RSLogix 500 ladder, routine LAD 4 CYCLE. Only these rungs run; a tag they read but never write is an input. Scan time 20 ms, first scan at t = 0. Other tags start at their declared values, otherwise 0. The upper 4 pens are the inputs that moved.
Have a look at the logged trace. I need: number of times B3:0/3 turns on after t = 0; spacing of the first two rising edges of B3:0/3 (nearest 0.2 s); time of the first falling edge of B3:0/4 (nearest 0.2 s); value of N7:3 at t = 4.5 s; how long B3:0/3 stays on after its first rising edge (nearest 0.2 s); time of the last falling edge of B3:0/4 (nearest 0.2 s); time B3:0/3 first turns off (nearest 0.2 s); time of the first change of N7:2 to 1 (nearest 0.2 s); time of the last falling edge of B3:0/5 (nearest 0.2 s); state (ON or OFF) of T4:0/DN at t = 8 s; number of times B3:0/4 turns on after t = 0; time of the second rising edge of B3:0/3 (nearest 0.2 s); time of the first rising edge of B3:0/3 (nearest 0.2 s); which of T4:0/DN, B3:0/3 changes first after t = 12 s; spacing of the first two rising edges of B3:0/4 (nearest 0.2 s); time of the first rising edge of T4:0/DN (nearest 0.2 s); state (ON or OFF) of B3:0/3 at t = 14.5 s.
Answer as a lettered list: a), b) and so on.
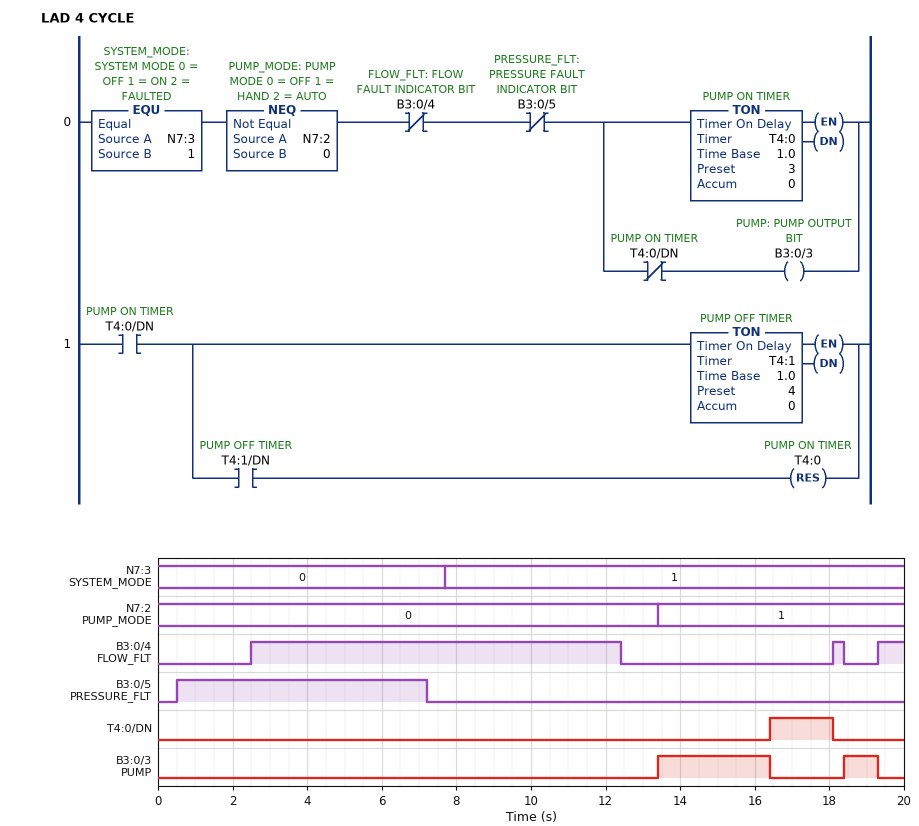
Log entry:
a) 2
b) 5.0 s
c) 12.4 s
d) 0
e) 3.0 s
f) 18.4 s
g) 16.4 s
h) 13.4 s
i) 7.2 s
j) OFF
k) 3
l) 18.4 s
m) 13.4 s
n) B3:0/3
o) 15.6 s
p) 16.4 s
q) ON
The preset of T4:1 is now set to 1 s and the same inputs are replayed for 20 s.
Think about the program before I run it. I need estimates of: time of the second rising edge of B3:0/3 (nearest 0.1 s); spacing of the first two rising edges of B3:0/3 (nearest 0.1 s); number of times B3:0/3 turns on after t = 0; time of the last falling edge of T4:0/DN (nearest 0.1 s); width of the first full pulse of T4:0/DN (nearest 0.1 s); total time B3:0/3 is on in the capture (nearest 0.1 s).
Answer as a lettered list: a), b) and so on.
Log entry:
a) 17.4 s
b) 4.0 s
c) 3
d) 17.4 s
e) 1.0 s
f) 4.6 s
